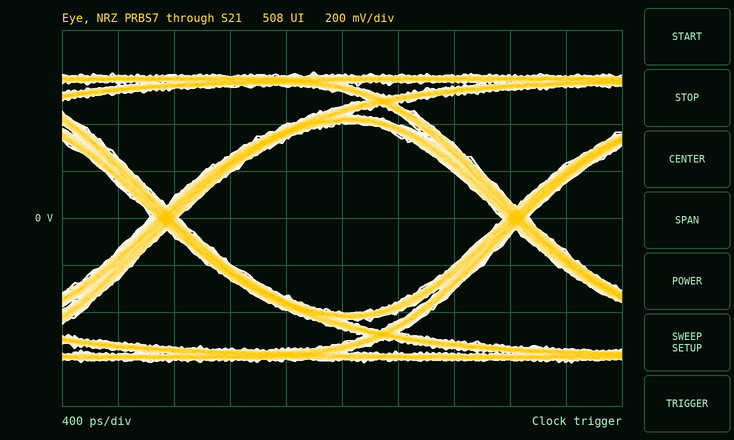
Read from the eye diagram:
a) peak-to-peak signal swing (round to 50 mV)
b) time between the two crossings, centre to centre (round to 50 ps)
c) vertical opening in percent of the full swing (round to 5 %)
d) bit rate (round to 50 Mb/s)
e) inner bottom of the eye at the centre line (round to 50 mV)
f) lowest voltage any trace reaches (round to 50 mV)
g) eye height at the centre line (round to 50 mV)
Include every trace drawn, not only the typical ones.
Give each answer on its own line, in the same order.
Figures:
1.25 V
2.50 ns
65 %
400 Mb/s
-400 mV
-600 mV
800 mV
